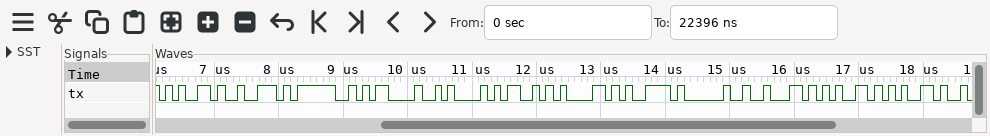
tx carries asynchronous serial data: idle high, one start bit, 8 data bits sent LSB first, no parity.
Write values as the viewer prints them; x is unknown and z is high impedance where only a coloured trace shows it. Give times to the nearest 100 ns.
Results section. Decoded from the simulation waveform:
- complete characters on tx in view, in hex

65, 72, 3F, 0D, 0A, 4D, 61, 79, 20, 62, 65, 65
